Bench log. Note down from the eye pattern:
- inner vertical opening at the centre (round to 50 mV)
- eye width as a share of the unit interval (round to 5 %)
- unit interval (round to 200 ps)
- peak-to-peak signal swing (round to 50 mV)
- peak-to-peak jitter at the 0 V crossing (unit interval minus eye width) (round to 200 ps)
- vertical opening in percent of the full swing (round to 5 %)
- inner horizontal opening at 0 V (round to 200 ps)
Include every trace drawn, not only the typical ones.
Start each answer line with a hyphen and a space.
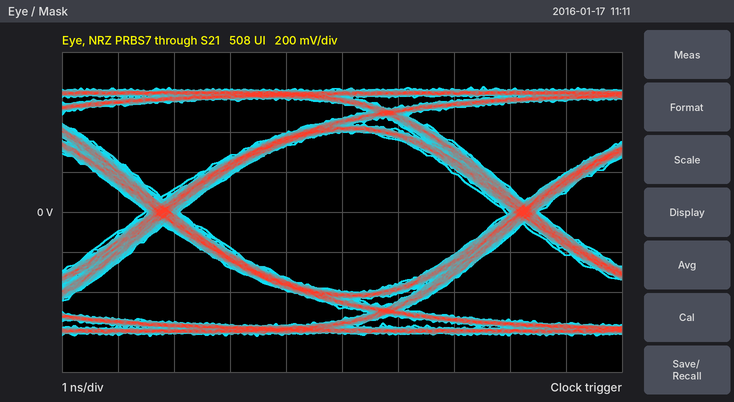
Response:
- 800 mV
- 90 %
- 6.4 ns
- 1.25 V
- 600 ps
- 65 %
- 5.8 ns
